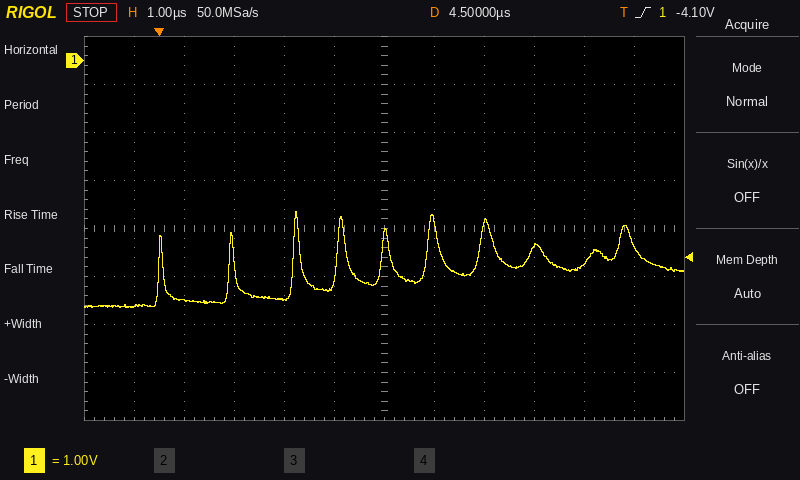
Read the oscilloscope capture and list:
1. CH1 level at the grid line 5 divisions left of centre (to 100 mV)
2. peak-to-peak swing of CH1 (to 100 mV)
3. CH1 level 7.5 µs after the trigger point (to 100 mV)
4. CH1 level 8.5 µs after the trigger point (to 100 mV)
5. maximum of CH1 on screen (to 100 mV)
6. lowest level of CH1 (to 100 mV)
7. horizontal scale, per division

-5.1 V
2.0 V
-3.9 V
-4.2 V
-3.1 V
-5.1 V
1 µs
